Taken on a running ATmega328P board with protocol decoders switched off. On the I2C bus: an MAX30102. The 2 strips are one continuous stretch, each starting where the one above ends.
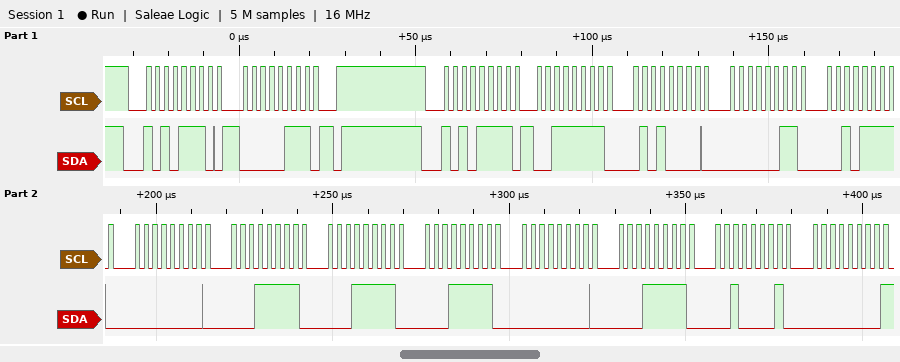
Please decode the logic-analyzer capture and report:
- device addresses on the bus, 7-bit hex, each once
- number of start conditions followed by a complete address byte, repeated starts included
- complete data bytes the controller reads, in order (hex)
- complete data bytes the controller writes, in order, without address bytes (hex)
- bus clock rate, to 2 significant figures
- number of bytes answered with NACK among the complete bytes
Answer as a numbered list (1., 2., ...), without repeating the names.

1. 0x57
2. 2
3. 3F 50 03 2F 00 1F 1F 1F 00 1F 21 00
4. 07
5. 400 kHz
6. 1
